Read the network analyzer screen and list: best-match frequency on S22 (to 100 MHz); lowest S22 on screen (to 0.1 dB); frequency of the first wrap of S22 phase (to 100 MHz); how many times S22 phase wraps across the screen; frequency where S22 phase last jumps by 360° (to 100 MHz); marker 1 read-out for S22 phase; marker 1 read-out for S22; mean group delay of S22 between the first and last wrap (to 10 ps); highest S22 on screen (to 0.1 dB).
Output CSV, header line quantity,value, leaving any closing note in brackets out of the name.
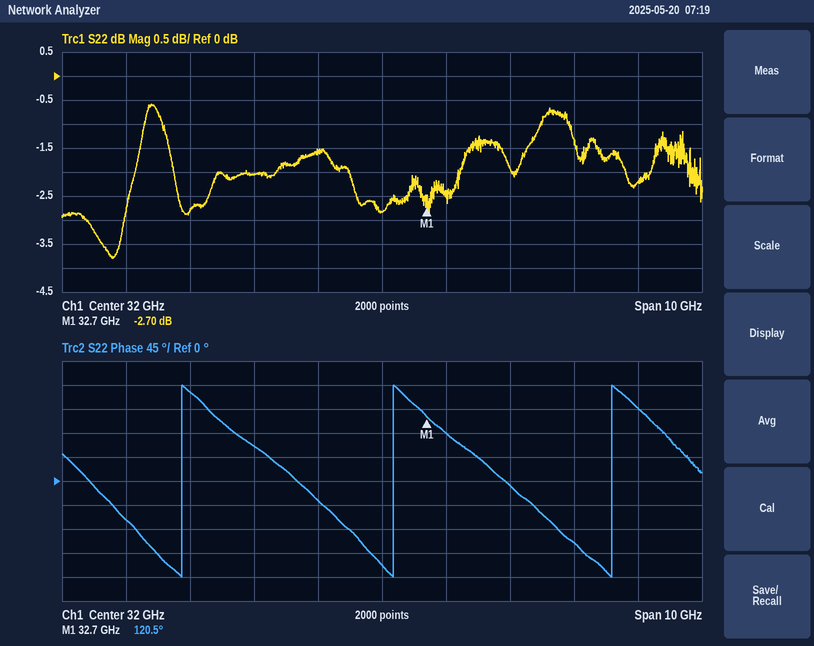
quantity,value
best-match frequency on S22,27.8 GHz
lowest S22 on screen,-3.8 dB
frequency of the first wrap of S22 phase,28.9 GHz
how many times S22 phase wraps across the screen,3
frequency where S22 phase last jumps by 360°,35.6 GHz
marker 1 read-out for S22 phase,120.5°
marker 1 read-out for S22,-2.70 dB
mean group delay of S22 between the first and last wrap,300 ps
highest S22 on screen,-0.6 dB
